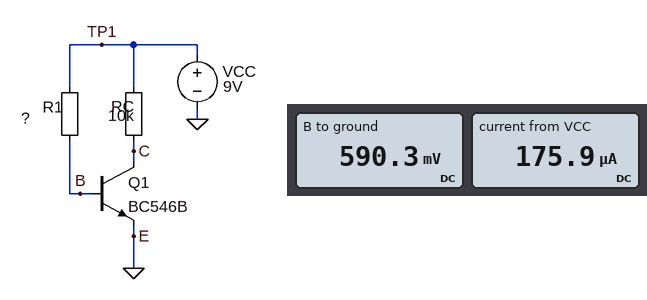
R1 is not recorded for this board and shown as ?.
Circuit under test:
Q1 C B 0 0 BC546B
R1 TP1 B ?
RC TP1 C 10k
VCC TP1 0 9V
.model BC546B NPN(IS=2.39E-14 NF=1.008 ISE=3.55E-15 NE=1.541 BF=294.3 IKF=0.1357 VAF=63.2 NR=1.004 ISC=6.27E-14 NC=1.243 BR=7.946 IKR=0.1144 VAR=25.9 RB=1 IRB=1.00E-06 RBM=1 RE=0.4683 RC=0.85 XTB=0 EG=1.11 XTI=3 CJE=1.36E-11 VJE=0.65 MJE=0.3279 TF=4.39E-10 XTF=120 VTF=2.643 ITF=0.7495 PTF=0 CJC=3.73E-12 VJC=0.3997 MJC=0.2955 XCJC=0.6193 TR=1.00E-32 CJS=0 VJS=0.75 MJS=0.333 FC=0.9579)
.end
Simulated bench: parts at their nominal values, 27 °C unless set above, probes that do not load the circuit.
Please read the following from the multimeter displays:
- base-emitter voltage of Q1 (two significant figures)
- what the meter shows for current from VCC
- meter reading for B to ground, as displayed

590 mV
175.9 µA
590.3 mV
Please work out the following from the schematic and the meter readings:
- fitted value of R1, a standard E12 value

15 MΩ
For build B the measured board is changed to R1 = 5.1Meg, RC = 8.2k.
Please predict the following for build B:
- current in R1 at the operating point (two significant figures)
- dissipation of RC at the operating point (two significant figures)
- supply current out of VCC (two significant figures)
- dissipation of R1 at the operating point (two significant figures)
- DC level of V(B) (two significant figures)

1.6 µA
2.0 mW
500 µA
14 µW
620 mV
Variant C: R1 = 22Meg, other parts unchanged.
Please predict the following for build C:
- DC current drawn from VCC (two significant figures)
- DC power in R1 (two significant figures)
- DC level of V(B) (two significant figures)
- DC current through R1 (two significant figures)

120 µA
3.2 µW
580 mV
380 nA
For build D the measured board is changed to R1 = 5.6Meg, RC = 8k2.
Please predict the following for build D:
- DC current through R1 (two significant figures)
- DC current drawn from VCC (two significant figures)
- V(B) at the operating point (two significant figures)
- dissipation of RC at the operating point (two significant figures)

1.5 µA
460 µA
620 mV
1.7 mW
